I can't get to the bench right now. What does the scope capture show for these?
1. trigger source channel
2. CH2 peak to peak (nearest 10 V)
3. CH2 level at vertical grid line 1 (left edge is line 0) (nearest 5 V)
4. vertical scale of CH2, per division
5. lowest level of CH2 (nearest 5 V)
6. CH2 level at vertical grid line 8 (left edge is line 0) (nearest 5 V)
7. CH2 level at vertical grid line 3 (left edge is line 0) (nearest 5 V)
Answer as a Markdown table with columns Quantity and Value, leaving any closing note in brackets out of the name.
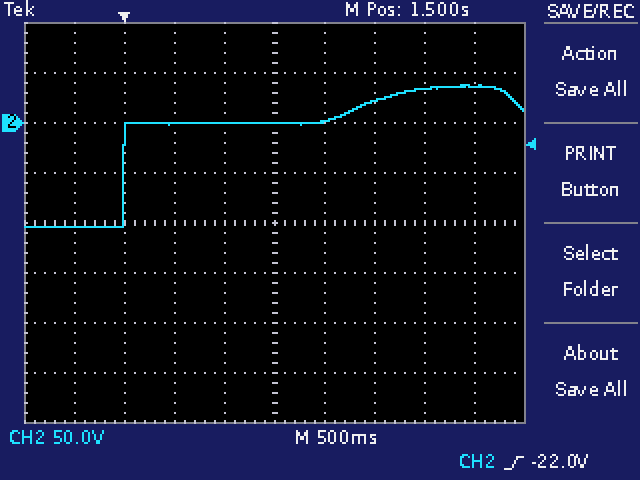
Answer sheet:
| Quantity | Value |
|---|---|
| trigger source channel | CH2 |
| CH2 peak to peak | 140 V |
| CH2 level at vertical grid line 1 (left edge is line 0) | -105 V |
| vertical scale of CH2, per division | 50 V |
| lowest level of CH2 | -105 V |
| CH2 level at vertical grid line 8 (left edge is line 0) | 35 V |
| CH2 level at vertical grid line 3 (left edge is line 0) | 0 V |
